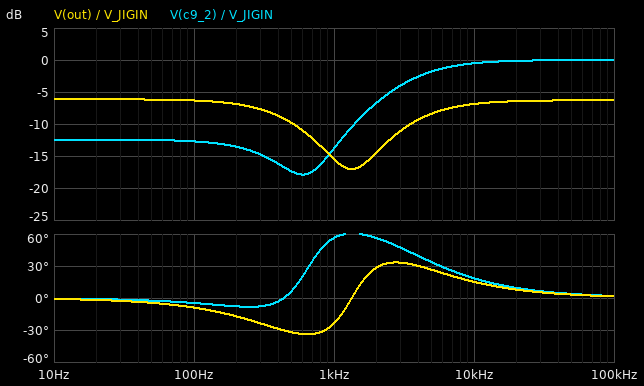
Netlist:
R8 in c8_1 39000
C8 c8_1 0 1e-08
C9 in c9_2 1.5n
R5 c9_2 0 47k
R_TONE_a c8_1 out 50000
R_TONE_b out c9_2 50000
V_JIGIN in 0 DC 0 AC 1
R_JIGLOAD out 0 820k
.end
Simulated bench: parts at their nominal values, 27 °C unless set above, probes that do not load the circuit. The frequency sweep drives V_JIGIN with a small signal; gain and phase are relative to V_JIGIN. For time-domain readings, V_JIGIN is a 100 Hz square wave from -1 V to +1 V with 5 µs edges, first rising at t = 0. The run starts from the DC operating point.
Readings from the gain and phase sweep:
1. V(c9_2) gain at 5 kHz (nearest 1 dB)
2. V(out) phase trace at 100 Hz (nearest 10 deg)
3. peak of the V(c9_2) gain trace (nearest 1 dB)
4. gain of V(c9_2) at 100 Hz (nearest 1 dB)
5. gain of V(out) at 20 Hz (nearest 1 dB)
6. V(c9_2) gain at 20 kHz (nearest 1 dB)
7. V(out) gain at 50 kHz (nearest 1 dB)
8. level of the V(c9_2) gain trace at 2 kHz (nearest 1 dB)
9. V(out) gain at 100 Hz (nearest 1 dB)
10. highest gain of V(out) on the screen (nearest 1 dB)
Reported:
-2 dB
-10 deg
0 dB
-13 dB
-6 dB
0 dB
-6 dB
-7 dB
-6 dB
-6 dB
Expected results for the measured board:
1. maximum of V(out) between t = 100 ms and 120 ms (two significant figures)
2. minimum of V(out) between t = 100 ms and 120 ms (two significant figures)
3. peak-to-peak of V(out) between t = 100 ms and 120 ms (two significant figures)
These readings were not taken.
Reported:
490 mV
-490 mV
990 mV
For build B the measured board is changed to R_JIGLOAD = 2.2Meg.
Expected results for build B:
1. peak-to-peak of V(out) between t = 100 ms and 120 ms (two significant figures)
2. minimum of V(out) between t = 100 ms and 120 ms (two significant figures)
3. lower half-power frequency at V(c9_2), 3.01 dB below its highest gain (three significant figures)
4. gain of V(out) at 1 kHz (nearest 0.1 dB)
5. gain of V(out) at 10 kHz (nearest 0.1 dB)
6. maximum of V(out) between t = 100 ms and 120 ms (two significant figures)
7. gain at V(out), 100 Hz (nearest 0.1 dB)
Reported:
1.0 V
-510 mV
3.61 kHz
-15.3 dB
-6.7 dB
510 mV
-6.0 dB
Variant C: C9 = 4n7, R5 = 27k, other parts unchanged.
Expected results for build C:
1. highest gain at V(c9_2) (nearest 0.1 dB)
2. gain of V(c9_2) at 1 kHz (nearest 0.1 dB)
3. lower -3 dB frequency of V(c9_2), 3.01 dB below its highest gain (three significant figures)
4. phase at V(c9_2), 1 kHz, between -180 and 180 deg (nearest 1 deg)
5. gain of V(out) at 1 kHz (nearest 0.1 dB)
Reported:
0 dB
-6.4 dB
1.76 kHz
53 deg
-11.8 dB
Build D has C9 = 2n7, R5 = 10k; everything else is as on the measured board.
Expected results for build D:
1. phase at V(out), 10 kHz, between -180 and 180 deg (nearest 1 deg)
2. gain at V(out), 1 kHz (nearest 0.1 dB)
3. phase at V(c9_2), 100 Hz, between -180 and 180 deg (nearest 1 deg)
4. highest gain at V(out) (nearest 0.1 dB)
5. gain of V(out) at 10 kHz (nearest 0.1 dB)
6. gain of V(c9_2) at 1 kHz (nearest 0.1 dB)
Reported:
30 deg
-17.0 dB
3 deg
-6.3 dB
-8.0 dB
-17.9 dB
